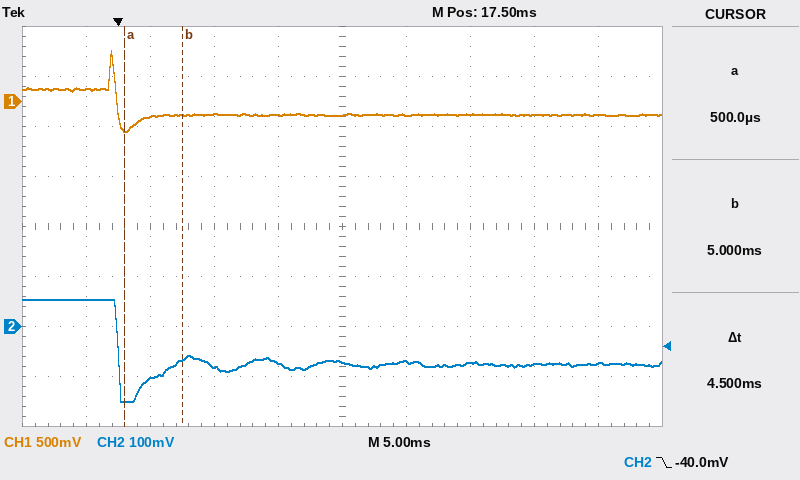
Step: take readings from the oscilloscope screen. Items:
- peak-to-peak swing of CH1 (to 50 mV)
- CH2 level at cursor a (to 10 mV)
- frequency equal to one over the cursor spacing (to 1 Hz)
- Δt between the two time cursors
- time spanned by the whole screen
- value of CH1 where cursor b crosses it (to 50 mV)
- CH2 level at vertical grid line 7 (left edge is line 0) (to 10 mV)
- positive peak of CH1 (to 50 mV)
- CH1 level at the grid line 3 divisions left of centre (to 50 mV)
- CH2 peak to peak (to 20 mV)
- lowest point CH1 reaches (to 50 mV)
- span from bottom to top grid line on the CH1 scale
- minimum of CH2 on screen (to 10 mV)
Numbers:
800 mV
-150 mV
222 Hz
4.5 ms
50 ms
-150 mV
-70 mV
500 mV
-150 mV
200 mV
-300 mV
4 V
-150 mV
